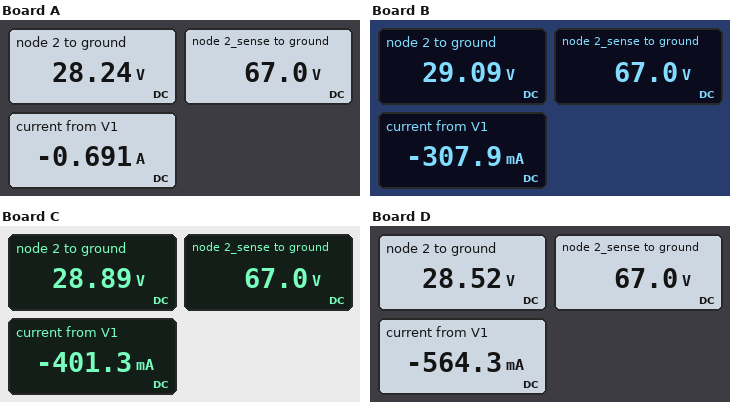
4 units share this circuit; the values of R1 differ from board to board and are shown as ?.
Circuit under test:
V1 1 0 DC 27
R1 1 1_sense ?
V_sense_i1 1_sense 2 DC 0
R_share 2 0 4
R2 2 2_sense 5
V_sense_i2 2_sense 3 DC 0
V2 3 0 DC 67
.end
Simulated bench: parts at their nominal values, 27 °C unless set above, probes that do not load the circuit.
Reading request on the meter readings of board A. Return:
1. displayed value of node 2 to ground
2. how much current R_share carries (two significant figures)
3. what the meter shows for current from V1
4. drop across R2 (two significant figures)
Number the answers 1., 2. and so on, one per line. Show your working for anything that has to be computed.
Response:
1. 28.24 V
2. (28.24 V) / 4 Ω = 7.1 A
3. -0.691 A
4. 67 V - 28.24 V = 39 V
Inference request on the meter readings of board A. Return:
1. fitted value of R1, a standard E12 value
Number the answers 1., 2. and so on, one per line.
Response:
1. 1.8 Ω
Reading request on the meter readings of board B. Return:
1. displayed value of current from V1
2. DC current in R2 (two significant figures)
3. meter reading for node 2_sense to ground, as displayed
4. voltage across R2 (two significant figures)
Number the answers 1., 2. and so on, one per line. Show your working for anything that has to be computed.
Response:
1. -307.9 mA
2. (67 V - 29.09 V) / 5 Ω = 7.6 A
3. 67.0 V
4. 67 V - 29.09 V = 38 V
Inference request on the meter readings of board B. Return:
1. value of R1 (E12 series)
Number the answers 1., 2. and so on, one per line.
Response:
1. 6.8 Ω
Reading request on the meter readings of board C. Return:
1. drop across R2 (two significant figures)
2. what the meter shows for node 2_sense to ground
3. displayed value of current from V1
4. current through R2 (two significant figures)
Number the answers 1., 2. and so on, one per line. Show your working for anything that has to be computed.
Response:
1. 67 V - 28.89 V = 38 V
2. 67.0 V
3. -401.3 mA
4. (67 V - 28.89 V) / 5 Ω = 7.6 A
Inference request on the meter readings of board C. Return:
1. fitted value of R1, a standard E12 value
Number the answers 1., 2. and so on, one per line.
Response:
1. 4.7 Ω
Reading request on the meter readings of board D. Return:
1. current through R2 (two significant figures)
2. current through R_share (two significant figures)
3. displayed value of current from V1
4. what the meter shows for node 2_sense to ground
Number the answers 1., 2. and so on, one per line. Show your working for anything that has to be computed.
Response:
1. (67 V - 28.52 V) / 5 Ω = 7.7 A
2. (28.52 V) / 4 Ω = 7.1 A
3. -564.3 mA
4. 67.0 V
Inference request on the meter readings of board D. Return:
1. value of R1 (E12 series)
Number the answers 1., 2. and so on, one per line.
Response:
1. 2.7 Ω
